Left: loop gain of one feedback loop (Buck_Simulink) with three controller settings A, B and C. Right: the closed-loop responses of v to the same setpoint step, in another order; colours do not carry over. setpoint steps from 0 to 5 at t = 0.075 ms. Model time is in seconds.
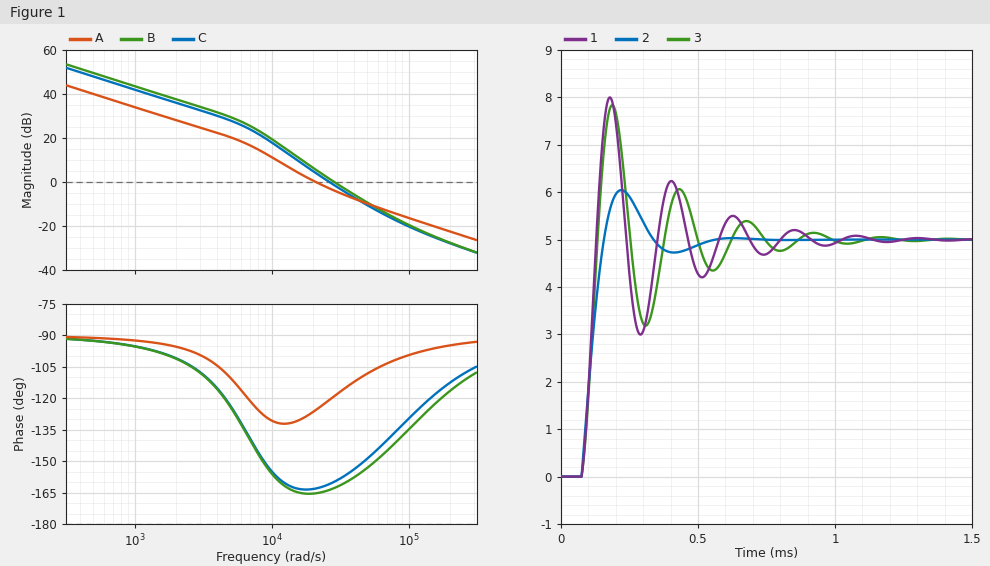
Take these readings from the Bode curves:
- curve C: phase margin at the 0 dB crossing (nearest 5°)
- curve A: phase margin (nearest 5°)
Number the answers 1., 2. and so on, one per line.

1. 20°
2. 55°
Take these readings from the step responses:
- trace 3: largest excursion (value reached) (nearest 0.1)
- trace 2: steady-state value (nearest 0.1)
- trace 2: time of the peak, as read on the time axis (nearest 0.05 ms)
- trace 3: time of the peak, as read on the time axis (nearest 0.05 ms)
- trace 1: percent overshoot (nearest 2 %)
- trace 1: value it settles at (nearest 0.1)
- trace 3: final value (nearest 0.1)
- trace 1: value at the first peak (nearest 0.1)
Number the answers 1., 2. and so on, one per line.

1. 7.8
2. 5.0
3. 0.20 ms
4. 0.20 ms
5. 60 %
6. 5.0
7. 5.0
8. 8.0
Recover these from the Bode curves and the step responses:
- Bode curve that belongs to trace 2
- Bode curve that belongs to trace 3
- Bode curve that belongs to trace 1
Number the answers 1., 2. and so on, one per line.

1. A
2. C
3. B
